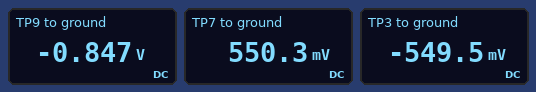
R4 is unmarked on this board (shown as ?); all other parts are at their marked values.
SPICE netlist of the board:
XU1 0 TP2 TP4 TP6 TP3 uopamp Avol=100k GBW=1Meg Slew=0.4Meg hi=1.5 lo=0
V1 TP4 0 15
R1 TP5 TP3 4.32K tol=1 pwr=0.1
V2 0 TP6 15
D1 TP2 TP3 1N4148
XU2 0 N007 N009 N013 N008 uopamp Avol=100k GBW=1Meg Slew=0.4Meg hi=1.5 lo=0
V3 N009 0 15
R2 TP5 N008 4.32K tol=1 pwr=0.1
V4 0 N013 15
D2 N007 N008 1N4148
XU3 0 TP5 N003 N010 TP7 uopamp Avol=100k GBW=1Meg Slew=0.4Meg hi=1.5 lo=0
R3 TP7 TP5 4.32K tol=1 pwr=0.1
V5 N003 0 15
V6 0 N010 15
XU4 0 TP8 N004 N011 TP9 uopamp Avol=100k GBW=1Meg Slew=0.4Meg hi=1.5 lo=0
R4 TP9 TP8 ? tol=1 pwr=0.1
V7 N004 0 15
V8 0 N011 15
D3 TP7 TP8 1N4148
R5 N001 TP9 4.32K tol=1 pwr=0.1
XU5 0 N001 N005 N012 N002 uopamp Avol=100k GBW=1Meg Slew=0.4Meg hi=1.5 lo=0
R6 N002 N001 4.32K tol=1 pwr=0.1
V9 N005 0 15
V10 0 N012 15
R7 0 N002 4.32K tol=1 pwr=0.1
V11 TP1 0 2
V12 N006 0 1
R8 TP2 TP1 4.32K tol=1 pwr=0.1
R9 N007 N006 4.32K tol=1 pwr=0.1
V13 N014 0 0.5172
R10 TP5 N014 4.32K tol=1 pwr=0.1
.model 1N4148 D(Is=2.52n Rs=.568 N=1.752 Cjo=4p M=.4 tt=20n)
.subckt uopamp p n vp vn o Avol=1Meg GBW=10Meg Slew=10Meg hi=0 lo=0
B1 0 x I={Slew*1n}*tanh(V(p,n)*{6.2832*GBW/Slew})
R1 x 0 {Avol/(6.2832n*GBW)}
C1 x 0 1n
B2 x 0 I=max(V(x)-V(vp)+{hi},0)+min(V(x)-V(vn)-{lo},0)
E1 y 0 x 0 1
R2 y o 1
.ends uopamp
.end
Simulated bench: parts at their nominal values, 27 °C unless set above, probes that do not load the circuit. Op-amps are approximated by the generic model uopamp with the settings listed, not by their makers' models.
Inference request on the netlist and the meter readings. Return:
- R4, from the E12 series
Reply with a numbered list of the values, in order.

1. 1.8 kΩ
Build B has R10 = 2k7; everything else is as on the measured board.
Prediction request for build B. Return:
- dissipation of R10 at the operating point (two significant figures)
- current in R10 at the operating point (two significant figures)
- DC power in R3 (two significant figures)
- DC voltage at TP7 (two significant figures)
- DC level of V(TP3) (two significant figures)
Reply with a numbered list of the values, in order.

1. 99 µW
2. 190 µA
3. 13 µW
4. 240 mV
5. -550 mV
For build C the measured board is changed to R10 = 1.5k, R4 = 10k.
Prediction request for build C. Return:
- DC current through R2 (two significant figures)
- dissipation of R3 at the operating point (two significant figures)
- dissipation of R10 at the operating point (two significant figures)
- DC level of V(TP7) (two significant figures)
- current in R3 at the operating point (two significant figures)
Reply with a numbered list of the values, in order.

1. 120 µA
2. 41 µW
3. 180 µW
4. -420 mV
5. 98 µA
